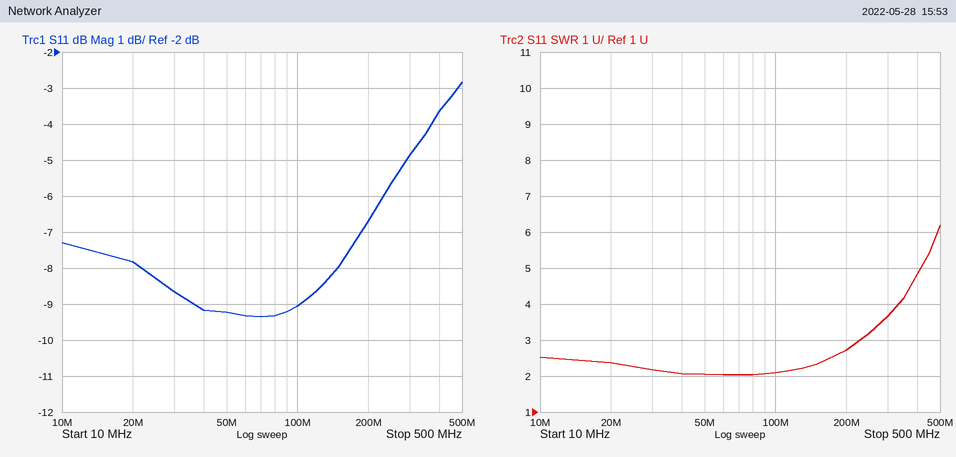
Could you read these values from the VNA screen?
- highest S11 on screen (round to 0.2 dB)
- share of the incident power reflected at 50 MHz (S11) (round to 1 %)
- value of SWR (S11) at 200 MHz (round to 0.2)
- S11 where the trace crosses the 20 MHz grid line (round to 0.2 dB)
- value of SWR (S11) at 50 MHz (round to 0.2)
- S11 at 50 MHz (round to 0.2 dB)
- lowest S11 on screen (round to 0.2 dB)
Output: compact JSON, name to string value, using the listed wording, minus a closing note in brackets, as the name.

{"highest S11 on screen": "-2.8 dB", "share of the incident power reflected at 50 MHz (S11)": "12 %", "value of SWR (S11) at 200 MHz": "2.8", "S11 where the trace crosses the 20 MHz grid line": "-7.8 dB", "value of SWR (S11) at 50 MHz": "2.0", "S11 at 50 MHz": "-9.2 dB", "lowest S11 on screen": "-9.4 dB"}
